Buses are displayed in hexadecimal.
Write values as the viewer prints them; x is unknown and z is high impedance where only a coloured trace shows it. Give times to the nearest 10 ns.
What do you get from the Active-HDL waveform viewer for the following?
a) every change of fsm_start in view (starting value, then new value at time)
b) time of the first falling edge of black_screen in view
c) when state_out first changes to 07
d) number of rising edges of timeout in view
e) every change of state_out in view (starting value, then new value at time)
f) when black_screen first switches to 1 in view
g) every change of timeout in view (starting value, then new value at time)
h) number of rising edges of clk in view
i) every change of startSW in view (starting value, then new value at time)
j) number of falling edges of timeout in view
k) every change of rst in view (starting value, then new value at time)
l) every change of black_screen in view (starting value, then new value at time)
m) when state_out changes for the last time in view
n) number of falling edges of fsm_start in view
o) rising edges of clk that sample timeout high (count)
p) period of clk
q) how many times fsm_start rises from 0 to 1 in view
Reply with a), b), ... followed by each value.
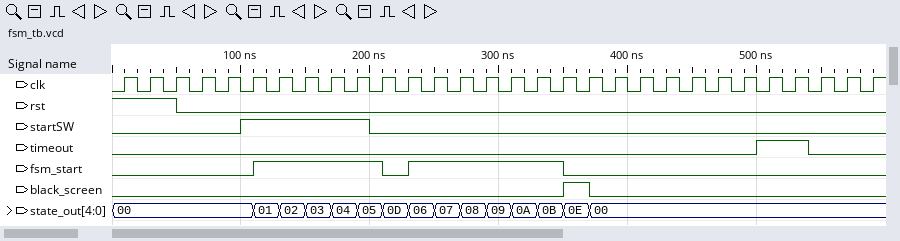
a) 0, 1 at 110 ns, 0 at 210 ns, 1 at 230 ns, 0 at 350 ns
b) 370 ns
c) 250 ns
d) 1
e) 00, 01 at 110 ns, 02 at 130 ns, 03 at 150 ns, 04 at 170 ns, 05 at 190 ns, 0D at 210 ns, 06 at 230 ns, 07 at 250 ns, 08 at 270 ns, 09 at 290 ns, 0A at 310 ns, 0B at 330 ns, 0E at 350 ns, 00 at 370 ns
f) 350 ns
g) 0, 1 at 500 ns, 0 at 540 ns
h) 30
i) 0, 1 at 100 ns, 0 at 200 ns
j) 1
k) 1, 0 at 50 ns
l) 0, 1 at 350 ns, 0 at 370 ns
m) 370 ns
n) 2
o) 2
p) 20 ns
q) 2
